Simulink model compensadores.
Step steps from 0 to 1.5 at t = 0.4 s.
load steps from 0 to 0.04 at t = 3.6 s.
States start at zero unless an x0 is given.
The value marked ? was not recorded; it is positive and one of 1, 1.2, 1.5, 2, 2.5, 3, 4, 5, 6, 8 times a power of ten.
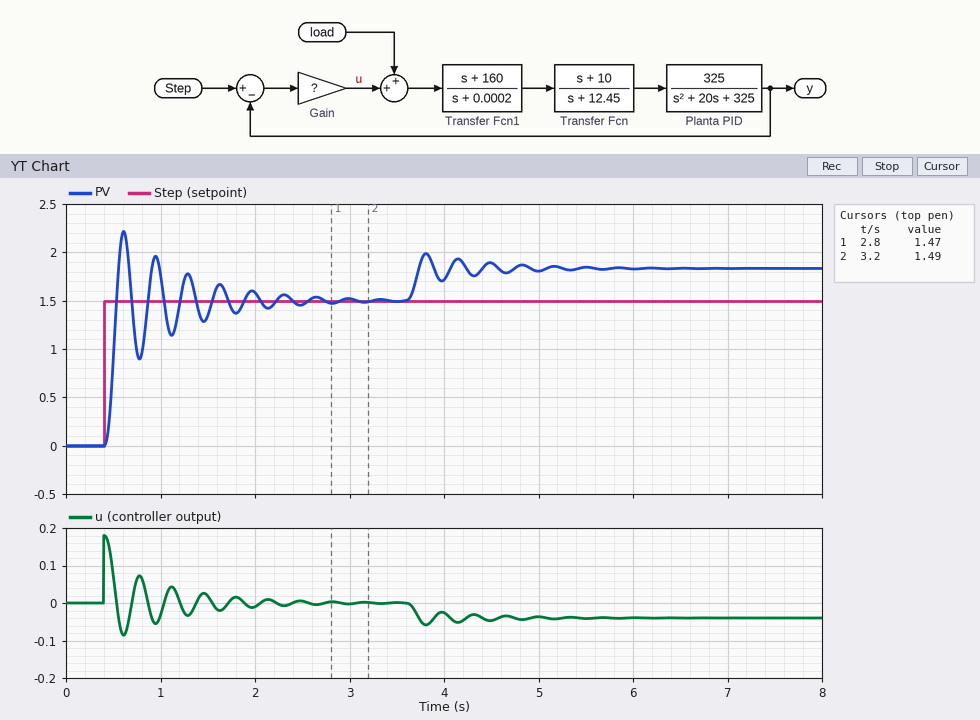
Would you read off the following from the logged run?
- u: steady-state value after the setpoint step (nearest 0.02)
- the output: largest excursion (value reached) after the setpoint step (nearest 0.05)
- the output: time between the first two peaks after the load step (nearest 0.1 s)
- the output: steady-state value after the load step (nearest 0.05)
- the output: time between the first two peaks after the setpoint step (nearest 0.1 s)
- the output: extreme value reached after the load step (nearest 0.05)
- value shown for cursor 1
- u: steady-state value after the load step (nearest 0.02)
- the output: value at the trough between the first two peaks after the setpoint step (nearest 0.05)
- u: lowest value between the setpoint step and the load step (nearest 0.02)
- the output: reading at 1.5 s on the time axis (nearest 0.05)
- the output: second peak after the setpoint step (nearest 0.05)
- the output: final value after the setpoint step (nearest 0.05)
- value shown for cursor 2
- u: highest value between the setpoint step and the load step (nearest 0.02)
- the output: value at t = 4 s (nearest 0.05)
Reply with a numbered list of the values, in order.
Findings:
1. 0.00
2. 2.20
3. 0.3 s
4. 1.85
5. 0.3 s
6. 2.00
7. 1.47
8. -0.04
9. 0.90
10. -0.08
11. 1.35
12. 1.95
13. 1.50
14. 1.49
15. 0.18
16. 1.70
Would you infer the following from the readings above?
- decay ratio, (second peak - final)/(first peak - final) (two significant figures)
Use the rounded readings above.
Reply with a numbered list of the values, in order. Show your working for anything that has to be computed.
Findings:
1. (1.95 - 1.5) / (2.2 - 1.5) = 0.64
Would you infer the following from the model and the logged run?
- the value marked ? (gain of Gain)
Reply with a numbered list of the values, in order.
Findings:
1. 0.12
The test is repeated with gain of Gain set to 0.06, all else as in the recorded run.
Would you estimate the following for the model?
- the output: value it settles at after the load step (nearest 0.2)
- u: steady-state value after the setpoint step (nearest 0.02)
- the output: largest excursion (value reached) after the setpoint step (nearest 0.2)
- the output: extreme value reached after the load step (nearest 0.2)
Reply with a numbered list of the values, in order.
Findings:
1. 2.2
2. 0.00
3. 1.6
4. 2.2
